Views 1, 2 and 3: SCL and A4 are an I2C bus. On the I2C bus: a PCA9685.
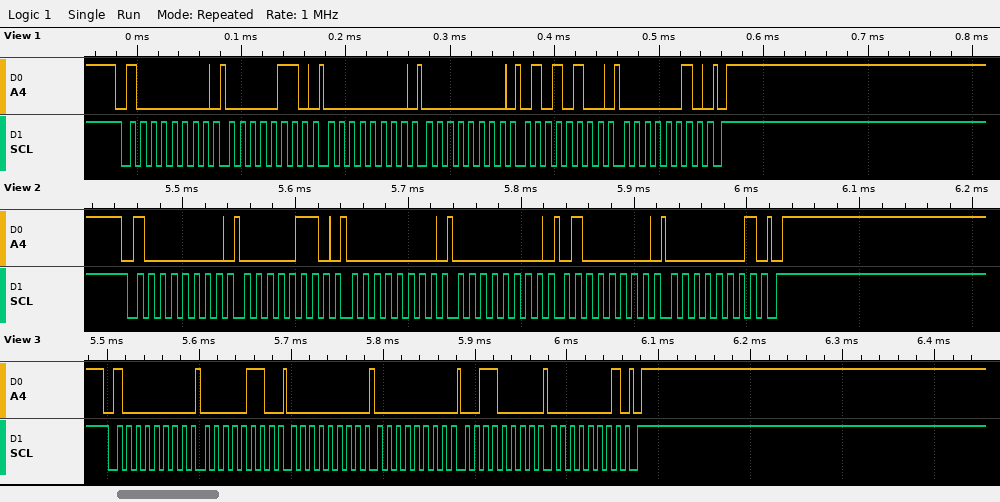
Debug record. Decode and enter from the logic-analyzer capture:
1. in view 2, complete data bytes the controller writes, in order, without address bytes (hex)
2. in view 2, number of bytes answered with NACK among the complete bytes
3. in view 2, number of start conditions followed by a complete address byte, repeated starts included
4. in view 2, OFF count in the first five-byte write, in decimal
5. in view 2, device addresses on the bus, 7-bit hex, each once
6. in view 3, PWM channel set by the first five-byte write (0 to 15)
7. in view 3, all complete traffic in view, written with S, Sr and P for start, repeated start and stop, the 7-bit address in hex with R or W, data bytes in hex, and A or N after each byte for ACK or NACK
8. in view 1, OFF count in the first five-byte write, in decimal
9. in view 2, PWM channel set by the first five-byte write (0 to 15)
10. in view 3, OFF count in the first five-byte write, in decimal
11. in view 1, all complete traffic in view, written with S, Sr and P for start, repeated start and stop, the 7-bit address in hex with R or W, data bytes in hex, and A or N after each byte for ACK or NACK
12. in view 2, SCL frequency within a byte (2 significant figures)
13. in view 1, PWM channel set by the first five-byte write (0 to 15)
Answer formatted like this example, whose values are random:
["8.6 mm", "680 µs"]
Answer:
["06 00 00 40 01", "0", "1", "320", "0x40", "0", "S 40W A 06 A 00 A 00 A 30 A 01 A P", "596", "0", "304", "S 40W A 06 A 00 A 00 A 54 A 02 A P", "100 kHz", "0"]
